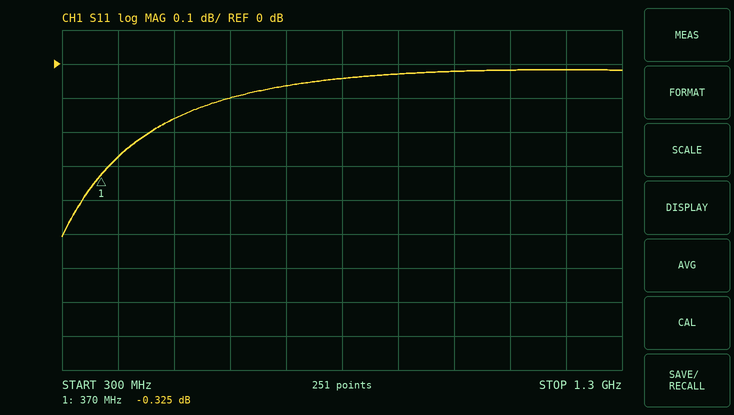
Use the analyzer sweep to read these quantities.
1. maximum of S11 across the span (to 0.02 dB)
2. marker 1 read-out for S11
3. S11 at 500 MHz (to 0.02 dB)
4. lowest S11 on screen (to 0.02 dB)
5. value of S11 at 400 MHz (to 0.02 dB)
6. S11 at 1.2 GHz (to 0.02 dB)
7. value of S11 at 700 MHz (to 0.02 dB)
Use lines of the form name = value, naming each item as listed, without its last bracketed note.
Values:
maximum of S11 across the span = -0.02 dB
marker 1 read-out for S11 = -0.325 dB
S11 at 500 MHz = -0.16 dB
lowest S11 on screen = -0.50 dB
value of S11 at 400 MHz = -0.28 dB
S11 at 1.2 GHz = -0.02 dB
value of S11 at 700 MHz = -0.06 dB
